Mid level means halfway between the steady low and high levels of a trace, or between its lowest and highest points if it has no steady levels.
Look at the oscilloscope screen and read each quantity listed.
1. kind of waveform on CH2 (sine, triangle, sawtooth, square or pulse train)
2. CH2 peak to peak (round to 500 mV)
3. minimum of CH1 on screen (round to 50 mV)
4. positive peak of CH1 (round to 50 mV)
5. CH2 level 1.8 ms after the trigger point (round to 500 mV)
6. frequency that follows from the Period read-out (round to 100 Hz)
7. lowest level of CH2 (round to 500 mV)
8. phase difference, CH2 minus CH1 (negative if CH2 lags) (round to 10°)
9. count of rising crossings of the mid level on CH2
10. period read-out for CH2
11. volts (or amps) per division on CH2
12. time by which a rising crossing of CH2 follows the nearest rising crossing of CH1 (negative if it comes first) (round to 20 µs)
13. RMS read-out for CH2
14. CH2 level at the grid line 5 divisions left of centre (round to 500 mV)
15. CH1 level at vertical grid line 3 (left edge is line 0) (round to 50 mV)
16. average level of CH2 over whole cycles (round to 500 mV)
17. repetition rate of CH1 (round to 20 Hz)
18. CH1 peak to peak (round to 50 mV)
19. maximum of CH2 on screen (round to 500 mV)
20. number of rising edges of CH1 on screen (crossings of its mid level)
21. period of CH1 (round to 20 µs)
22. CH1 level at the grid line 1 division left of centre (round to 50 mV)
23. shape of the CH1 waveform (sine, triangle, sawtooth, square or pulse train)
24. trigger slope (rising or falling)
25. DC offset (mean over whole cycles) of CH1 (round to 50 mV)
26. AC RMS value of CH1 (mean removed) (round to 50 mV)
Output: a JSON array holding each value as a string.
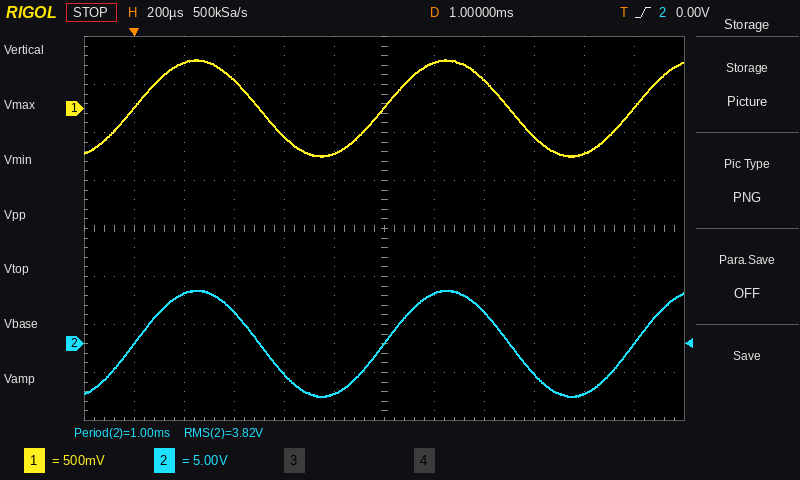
["sine", "11.0 V", "-500 mV", "500 mV", "-5.0 V", "1.0 kHz", "-5.5 V", "0°", "3", "1.00 ms", "5 V", "0 µs", "3.82 V", "0.0 V", "300 mV", "0.0 V", "1.00 kHz", "1.00 V", "5.5 V", "3", "1.00 ms", "-450 mV", "sine", "rising", "0 mV", "350 mV"]
